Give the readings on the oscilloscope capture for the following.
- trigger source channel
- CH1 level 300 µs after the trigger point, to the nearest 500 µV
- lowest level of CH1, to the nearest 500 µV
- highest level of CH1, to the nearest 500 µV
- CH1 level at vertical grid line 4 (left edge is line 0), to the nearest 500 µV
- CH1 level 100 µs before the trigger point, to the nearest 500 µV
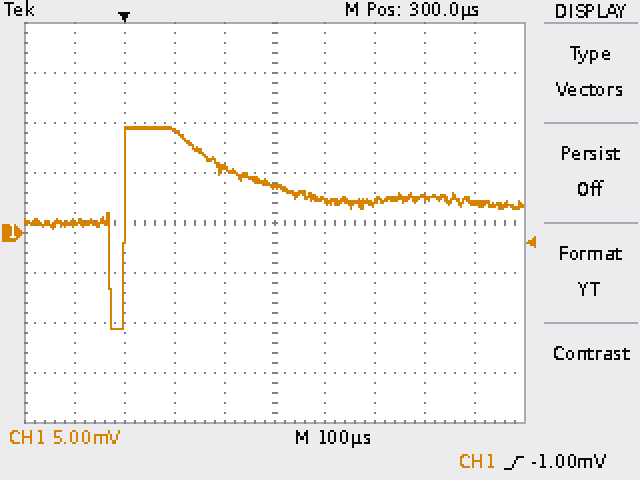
CH1
4.5 mV
-9.5 mV
10.5 mV
6.5 mV
1.0 mV
